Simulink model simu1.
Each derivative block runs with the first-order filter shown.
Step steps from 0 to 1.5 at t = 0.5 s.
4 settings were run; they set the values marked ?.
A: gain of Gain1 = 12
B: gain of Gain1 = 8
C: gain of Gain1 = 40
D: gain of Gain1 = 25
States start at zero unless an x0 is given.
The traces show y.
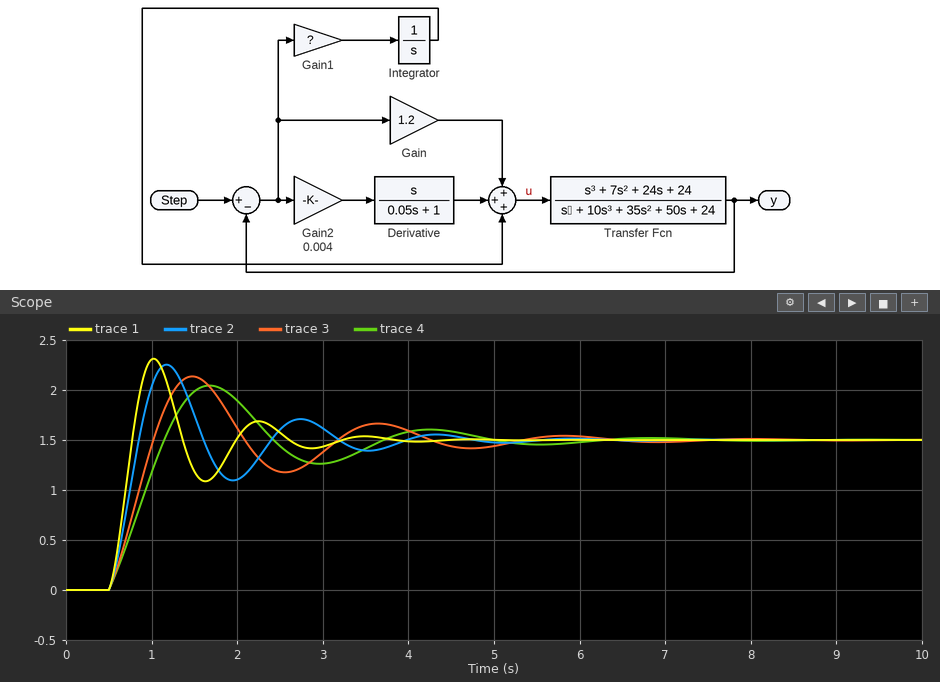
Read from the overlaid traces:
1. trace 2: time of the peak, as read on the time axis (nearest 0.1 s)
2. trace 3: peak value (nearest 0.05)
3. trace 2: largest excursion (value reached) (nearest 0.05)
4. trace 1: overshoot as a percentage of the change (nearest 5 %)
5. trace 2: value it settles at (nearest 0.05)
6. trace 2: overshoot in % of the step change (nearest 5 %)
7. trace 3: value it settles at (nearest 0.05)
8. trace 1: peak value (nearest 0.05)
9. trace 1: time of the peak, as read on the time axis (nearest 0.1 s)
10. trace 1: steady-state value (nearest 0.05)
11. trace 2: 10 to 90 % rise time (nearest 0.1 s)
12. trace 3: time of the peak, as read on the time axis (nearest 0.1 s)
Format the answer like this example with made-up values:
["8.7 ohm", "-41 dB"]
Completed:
["1.2 s", "2.15", "2.25", "55 %", "1.50", "50 %", "1.50", "2.30", "1.0 s", "1.50", "0.3 s", "1.5 s"]
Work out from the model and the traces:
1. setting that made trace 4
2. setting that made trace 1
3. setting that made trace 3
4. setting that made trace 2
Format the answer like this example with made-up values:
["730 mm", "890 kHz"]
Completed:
["B", "C", "A", "D"]
